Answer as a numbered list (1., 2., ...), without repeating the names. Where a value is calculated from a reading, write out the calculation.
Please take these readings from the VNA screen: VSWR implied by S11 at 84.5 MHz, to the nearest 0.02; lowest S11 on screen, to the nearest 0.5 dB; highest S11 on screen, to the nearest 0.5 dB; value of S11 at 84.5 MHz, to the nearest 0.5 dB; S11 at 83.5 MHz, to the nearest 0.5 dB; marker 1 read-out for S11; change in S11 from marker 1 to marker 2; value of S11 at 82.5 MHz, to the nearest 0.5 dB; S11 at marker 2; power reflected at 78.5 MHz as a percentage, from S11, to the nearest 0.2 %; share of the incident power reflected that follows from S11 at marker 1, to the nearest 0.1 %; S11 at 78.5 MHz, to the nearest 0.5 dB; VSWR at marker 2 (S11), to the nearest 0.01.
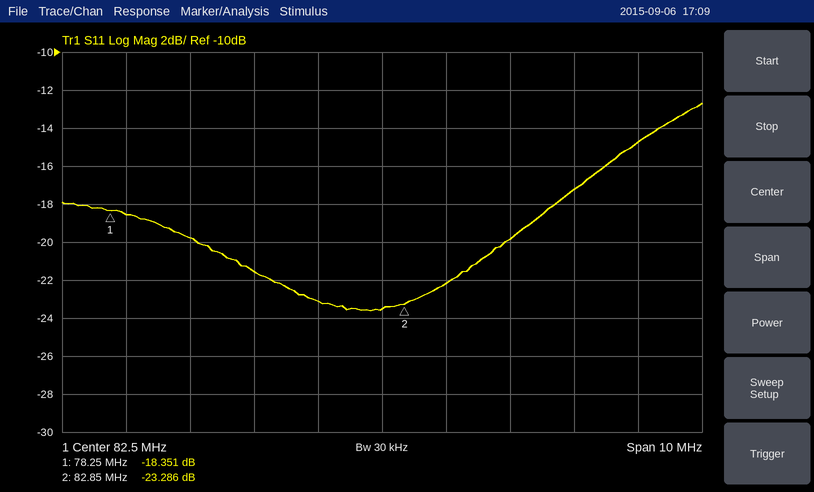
1. |Γ| = 10^(-20/20) = 0.1000; VSWR = (1 + 0.1000)/(1 − 0.1000) ≈ 1.22
2. -23.5 dB
3. -12.5 dB
4. -20.0 dB
5. -22.0 dB
6. -18.351 dB
7. -23.286 − (-18.351) = -4.935 dB
8. -23.5 dB
9. -23.286 dB
10. 10^(-18.5/10) ≈ 1.4 %
11. 10^(-18.351/10) ≈ 1.5 %
12. -18.5 dB
13. (1 + 0.0685)/(1 − 0.0685) ≈ 1.15
